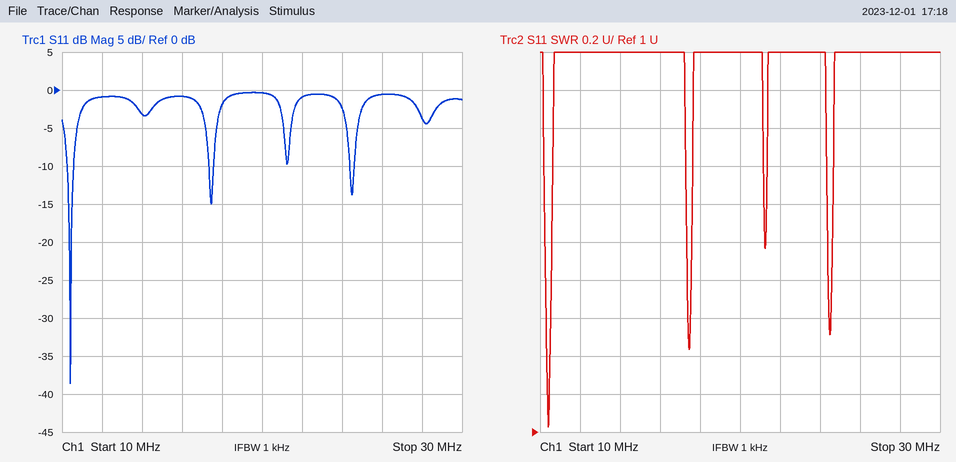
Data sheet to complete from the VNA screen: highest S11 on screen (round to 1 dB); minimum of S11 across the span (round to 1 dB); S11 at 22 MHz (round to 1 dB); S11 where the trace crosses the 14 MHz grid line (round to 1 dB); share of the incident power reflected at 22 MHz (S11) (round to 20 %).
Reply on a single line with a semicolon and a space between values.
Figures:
0 dB; -39 dB; -1 dB; -3 dB; 80 %
